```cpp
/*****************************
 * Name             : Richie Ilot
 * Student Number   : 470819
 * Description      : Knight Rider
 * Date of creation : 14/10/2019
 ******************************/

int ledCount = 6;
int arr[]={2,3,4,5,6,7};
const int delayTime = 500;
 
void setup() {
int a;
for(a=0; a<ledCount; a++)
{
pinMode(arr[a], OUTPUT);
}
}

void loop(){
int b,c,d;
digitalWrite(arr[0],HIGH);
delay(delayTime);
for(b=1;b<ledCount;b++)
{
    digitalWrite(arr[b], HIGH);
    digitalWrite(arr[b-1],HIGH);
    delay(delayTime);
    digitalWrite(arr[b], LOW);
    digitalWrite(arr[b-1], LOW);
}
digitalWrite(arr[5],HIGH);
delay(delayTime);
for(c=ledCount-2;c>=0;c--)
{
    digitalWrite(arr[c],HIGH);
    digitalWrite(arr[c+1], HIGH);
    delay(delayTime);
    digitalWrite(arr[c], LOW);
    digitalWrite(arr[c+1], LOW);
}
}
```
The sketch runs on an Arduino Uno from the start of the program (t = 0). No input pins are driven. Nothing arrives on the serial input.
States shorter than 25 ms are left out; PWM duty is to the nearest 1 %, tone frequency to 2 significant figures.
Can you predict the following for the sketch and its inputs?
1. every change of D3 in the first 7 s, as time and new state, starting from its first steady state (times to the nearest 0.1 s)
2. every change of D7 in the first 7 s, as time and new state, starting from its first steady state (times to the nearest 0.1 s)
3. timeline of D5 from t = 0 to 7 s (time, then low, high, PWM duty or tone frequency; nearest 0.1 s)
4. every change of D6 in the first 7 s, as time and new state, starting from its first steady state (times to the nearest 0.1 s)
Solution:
0 s low; 0.5 s high; 1.5 s low; 5 s high; 6 s low; 6.5 s high
0 s low; 2.5 s high; 4 s low
0 s low; 1.5 s high; 2.5 s low; 4 s high; 5 s low
0 s low; 2 s high; 3 s low; 3.5 s high; 4.5 s low
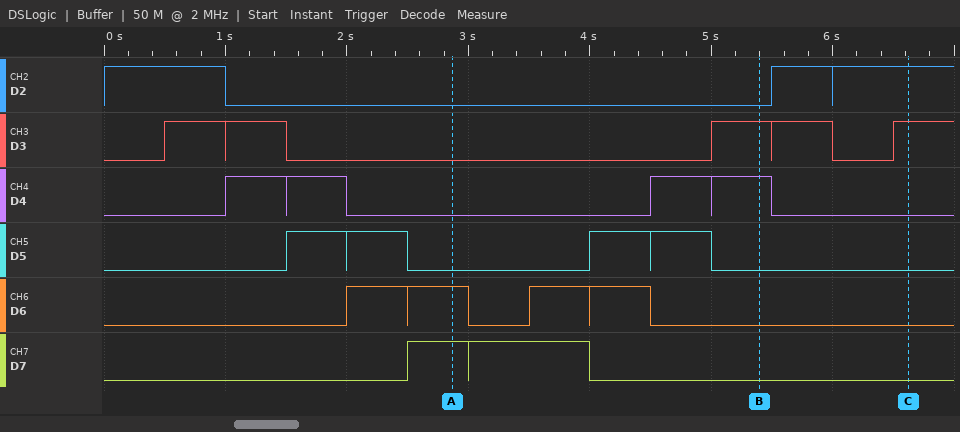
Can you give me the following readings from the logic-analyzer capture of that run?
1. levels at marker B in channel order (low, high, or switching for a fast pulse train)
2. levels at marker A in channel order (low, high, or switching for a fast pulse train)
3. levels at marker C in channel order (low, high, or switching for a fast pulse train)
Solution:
D2 low, D3 high, D4 high, D5 low, D6 low, D7 low
D2 low, D3 low, D4 low, D5 low, D6 high, D7 high
D2 high, D3 high, D4 low, D5 low, D6 low, D7 low
